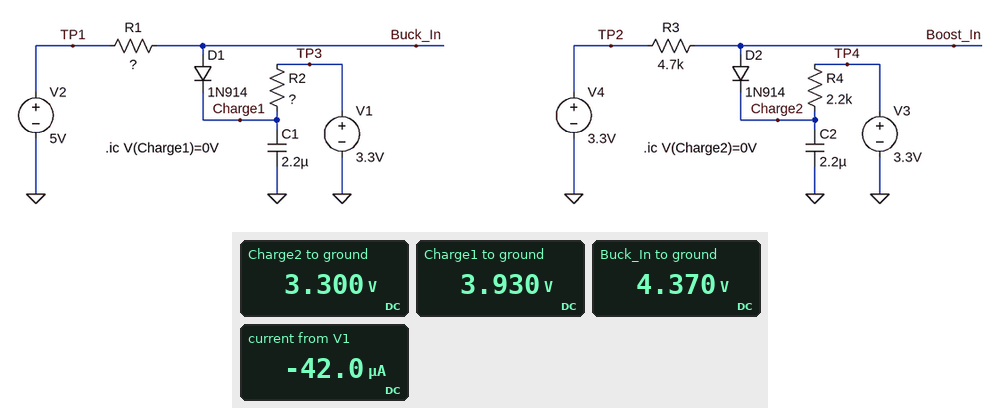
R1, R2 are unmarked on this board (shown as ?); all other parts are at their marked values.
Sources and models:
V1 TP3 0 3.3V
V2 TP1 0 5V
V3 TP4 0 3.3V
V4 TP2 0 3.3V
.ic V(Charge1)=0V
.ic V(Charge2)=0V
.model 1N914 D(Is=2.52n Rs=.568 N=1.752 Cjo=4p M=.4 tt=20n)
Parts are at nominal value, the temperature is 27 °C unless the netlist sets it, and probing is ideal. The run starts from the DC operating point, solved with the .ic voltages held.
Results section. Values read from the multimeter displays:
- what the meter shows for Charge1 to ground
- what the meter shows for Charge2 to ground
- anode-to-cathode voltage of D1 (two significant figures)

3.930 V
3.300 V
440 mV
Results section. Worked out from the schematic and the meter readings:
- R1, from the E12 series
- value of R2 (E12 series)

15 kΩ
15 kΩ
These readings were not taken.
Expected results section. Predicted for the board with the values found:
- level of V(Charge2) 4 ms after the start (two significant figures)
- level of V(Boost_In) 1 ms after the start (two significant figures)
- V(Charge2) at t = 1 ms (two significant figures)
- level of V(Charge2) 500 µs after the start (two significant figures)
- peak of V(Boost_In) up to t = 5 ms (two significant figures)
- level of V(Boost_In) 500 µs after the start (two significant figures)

2.2 V
1.4 V
820 mV
440 mV
2.9 V
990 mV
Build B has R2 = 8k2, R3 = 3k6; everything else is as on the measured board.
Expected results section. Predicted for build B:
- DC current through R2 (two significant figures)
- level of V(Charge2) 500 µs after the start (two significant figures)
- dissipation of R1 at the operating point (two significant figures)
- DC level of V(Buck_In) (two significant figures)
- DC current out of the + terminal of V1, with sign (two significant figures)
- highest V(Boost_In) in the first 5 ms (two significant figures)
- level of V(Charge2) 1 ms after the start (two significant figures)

54 µA
470 mV
43 µW
4.2 V
-54 µA
3.0 V
870 mV
